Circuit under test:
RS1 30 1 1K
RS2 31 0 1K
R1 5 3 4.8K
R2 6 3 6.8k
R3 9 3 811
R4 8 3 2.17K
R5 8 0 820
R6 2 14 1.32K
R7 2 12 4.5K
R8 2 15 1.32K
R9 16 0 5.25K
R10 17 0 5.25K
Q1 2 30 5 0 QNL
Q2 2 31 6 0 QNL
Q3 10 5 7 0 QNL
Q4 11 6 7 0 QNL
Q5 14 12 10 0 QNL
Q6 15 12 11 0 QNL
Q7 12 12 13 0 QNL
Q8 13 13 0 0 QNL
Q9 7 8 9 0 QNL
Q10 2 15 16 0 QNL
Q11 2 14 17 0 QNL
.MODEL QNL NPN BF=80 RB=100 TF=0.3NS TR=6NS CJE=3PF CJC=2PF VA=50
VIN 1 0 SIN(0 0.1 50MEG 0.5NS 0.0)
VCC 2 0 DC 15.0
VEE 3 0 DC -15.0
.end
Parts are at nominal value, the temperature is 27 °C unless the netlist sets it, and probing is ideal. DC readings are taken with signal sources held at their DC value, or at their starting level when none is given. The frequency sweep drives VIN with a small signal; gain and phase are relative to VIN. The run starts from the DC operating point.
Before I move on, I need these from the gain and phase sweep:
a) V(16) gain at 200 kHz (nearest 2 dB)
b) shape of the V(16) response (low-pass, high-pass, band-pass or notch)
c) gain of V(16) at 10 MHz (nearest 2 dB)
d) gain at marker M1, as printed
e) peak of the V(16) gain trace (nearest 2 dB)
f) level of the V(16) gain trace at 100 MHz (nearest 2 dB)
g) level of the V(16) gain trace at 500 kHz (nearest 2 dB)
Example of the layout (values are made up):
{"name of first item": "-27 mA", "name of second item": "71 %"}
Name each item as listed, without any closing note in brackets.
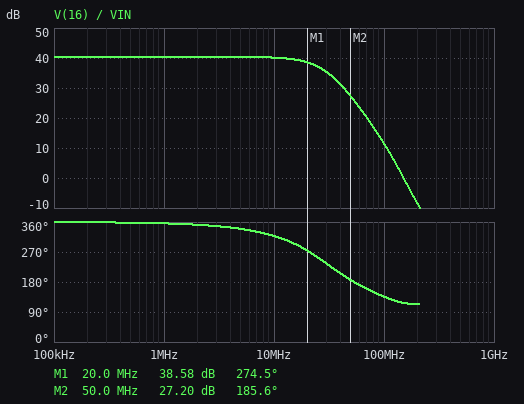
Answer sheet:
{"V(16) gain at 200 kHz": "40 dB", "shape of the V(16) response": "low-pass", "gain of V(16) at 10 MHz": "40 dB", "gain at marker M1, as printed": "38.58 dB", "peak of the V(16) gain trace": "40 dB", "level of the V(16) gain trace at 100 MHz": "12 dB", "level of the V(16) gain trace at 500 kHz": "40 dB"}
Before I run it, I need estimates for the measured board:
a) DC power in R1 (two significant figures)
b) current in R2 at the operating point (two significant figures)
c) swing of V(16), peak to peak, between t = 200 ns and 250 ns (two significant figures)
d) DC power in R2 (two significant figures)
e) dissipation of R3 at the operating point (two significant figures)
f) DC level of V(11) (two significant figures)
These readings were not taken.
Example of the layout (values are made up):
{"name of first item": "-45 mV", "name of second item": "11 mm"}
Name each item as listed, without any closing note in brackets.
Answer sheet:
{"DC power in R1": "42 mW", "current in R2 at the operating point": "2.1 mA", "swing of V(16), peak to peak, between t = 200 ns and 250 ns": "4.5 V", "DC power in R2": "30 mW", "dissipation of R3 at the operating point": "120 mW", "DC level of V(11)": "780 mV"}
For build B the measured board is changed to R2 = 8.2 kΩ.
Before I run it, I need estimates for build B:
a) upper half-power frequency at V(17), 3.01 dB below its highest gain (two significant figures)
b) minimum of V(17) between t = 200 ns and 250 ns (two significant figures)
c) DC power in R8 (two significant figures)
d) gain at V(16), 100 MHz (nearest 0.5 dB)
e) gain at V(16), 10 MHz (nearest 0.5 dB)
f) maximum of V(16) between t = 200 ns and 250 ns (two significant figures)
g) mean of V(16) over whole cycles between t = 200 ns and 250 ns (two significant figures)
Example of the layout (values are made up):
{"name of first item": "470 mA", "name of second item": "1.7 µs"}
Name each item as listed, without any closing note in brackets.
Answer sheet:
{"upper half-power frequency at V(17), 3.01 dB below its highest gain": "25 MHz", "minimum of V(17) between t = 200 ns and 250 ns": "6.7 V", "DC power in R8": "86 mW", "gain at V(16), 100 MHz": "11.0 dB", "gain at V(16), 10 MHz": "39.5 dB", "maximum of V(16) between t = 200 ns and 250 ns": "6.0 V", "mean of V(16) over whole cycles between t = 200 ns and 250 ns": "3.8 V"}
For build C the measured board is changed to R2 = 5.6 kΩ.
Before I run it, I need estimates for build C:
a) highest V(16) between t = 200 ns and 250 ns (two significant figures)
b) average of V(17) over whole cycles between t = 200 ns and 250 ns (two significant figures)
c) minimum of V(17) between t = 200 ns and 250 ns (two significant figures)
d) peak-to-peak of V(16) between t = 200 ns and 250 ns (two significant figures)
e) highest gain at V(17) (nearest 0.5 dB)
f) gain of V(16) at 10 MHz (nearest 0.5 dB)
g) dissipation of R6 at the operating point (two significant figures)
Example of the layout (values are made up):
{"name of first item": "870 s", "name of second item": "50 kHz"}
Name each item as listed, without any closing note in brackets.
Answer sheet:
{"highest V(16) between t = 200 ns and 250 ns": "7.9 V", "average of V(17) over whole cycles between t = 200 ns and 250 ns": "7.3 V", "minimum of V(17) between t = 200 ns and 250 ns": "4.9 V", "peak-to-peak of V(16) between t = 200 ns and 250 ns": "4.7 V", "highest gain at V(17)": "41.0 dB", "gain of V(16) at 10 MHz": "40.5 dB", "dissipation of R6 at the operating point": "36 mW"}
